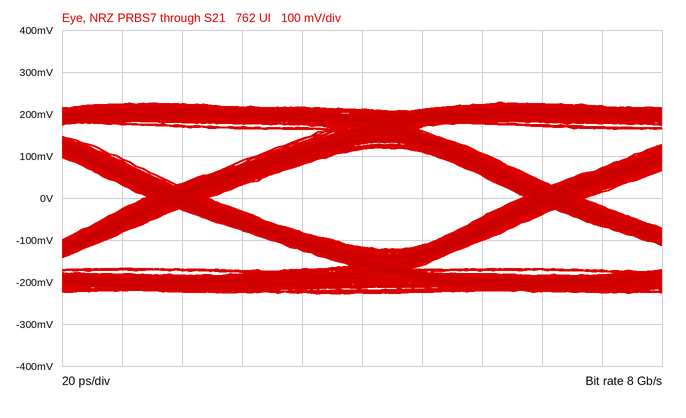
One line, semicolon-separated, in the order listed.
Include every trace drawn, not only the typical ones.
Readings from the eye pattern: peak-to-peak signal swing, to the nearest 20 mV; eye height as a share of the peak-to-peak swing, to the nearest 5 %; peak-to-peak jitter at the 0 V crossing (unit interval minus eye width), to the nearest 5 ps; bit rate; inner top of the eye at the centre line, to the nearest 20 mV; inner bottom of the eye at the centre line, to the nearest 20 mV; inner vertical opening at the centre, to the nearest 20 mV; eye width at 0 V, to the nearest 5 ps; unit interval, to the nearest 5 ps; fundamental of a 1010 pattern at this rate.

460 mV; 50 %; 20 ps; 8 Gb/s; 120 mV; -120 mV; 240 mV; 105 ps; 125 ps; 4 GHz
